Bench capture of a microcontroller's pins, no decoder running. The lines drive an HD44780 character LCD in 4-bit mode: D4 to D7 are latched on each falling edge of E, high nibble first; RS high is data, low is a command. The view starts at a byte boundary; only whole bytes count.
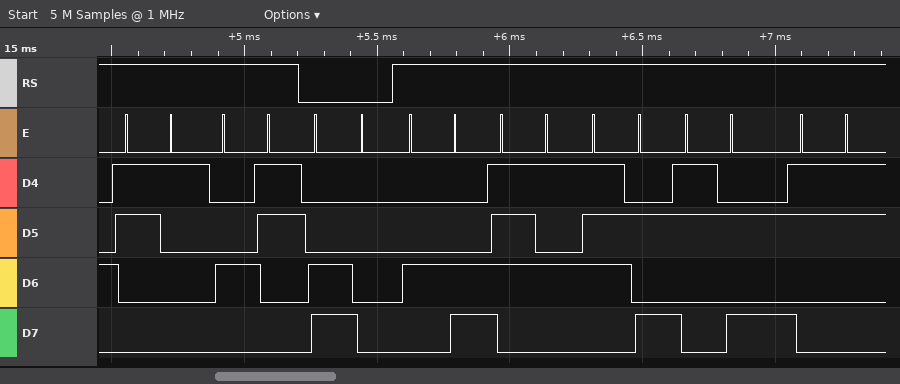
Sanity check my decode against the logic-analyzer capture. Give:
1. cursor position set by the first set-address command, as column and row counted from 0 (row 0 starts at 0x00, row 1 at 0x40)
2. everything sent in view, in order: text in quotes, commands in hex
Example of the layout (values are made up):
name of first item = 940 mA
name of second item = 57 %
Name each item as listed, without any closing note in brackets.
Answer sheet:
cursor position set by the first set-address command, as column and row counted from 0 = column 0, row 1
everything sent in view, in order: text in quotes, commands in hex = "1C" 0xC0 "Luz:3"
